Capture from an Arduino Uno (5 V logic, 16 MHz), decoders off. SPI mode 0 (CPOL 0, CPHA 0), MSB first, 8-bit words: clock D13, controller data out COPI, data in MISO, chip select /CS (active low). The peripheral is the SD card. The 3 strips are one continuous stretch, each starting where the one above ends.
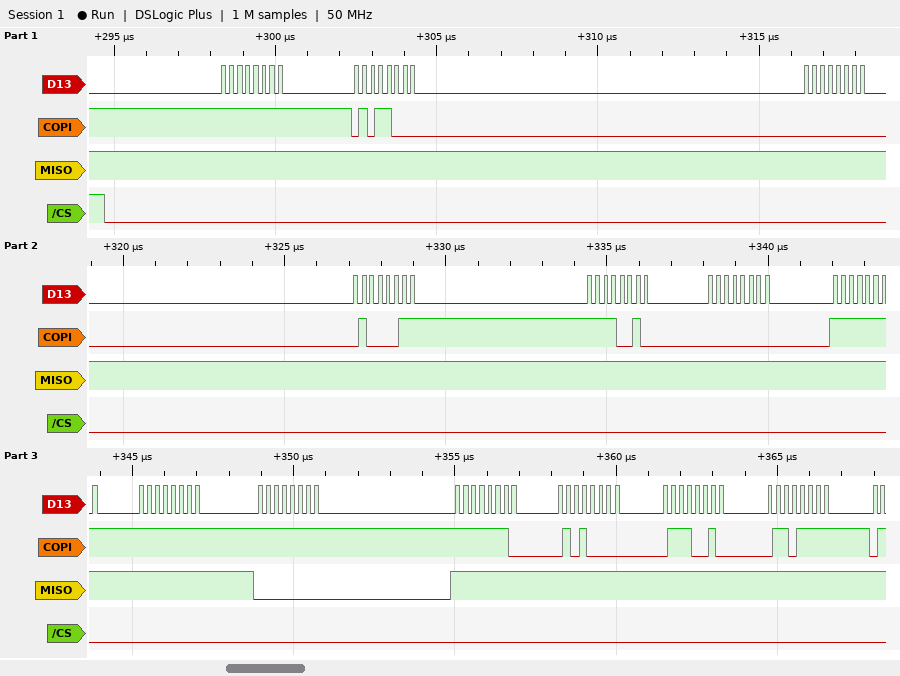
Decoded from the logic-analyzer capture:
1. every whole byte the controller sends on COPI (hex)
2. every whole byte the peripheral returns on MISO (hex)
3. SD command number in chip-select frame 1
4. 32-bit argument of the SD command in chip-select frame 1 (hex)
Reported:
FF 58 00 43 F2 00 FF FF FF FE 50 72 6F
FF FF FF FF FF FF FF FF 00 FF FF FF FF
CMD24
0x0043F200
